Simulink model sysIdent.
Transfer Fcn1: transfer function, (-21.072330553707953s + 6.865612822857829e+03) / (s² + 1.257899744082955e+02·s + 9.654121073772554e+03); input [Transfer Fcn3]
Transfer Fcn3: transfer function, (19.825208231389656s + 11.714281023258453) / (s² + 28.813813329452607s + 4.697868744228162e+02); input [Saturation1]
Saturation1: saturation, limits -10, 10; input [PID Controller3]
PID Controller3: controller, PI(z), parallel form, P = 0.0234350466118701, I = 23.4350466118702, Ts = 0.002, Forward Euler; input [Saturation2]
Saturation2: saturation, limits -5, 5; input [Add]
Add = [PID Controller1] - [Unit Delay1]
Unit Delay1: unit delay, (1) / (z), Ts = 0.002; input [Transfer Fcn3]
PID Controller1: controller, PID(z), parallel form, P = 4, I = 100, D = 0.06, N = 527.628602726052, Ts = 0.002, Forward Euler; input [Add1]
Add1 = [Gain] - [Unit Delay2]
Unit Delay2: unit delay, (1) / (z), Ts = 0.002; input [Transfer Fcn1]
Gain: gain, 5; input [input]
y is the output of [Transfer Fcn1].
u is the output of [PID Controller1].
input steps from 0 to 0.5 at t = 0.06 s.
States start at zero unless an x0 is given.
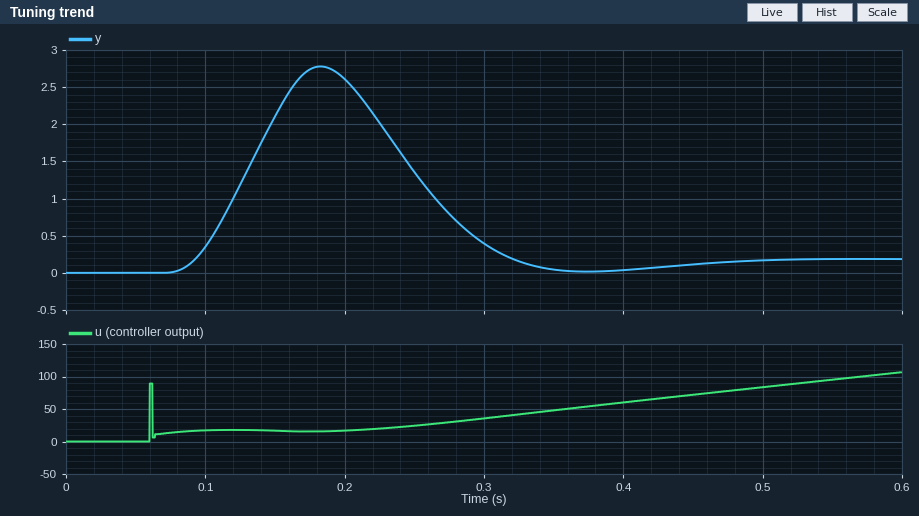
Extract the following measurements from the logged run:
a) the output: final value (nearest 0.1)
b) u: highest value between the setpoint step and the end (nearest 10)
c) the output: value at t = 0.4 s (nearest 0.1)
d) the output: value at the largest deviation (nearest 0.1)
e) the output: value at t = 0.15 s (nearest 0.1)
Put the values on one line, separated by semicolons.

0.2; 110; 0.0; 2.8; 2.1
